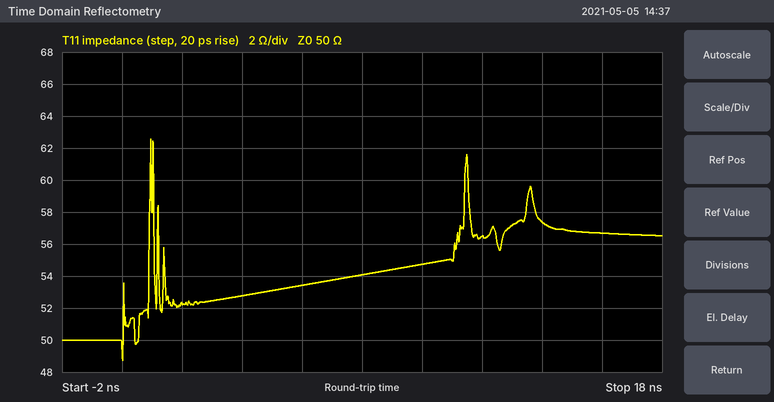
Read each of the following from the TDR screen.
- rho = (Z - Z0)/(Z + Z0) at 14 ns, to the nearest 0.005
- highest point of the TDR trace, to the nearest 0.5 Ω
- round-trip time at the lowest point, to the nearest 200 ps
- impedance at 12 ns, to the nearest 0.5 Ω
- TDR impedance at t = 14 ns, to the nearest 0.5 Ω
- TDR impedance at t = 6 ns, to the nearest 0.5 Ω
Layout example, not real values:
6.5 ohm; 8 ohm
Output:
+0.070; 62.5 Ω; 0.0 ns; 56.5 Ω; 57.5 Ω; 53.5 Ω
